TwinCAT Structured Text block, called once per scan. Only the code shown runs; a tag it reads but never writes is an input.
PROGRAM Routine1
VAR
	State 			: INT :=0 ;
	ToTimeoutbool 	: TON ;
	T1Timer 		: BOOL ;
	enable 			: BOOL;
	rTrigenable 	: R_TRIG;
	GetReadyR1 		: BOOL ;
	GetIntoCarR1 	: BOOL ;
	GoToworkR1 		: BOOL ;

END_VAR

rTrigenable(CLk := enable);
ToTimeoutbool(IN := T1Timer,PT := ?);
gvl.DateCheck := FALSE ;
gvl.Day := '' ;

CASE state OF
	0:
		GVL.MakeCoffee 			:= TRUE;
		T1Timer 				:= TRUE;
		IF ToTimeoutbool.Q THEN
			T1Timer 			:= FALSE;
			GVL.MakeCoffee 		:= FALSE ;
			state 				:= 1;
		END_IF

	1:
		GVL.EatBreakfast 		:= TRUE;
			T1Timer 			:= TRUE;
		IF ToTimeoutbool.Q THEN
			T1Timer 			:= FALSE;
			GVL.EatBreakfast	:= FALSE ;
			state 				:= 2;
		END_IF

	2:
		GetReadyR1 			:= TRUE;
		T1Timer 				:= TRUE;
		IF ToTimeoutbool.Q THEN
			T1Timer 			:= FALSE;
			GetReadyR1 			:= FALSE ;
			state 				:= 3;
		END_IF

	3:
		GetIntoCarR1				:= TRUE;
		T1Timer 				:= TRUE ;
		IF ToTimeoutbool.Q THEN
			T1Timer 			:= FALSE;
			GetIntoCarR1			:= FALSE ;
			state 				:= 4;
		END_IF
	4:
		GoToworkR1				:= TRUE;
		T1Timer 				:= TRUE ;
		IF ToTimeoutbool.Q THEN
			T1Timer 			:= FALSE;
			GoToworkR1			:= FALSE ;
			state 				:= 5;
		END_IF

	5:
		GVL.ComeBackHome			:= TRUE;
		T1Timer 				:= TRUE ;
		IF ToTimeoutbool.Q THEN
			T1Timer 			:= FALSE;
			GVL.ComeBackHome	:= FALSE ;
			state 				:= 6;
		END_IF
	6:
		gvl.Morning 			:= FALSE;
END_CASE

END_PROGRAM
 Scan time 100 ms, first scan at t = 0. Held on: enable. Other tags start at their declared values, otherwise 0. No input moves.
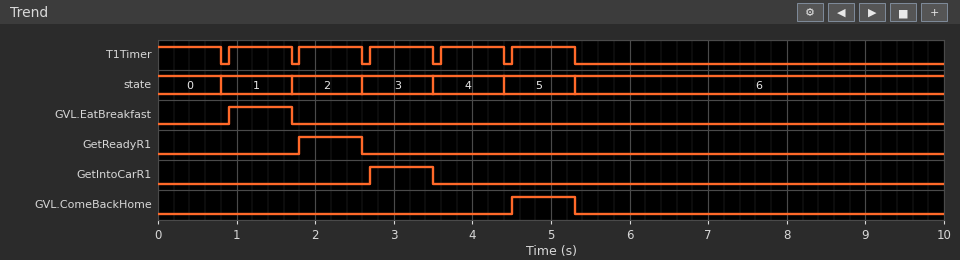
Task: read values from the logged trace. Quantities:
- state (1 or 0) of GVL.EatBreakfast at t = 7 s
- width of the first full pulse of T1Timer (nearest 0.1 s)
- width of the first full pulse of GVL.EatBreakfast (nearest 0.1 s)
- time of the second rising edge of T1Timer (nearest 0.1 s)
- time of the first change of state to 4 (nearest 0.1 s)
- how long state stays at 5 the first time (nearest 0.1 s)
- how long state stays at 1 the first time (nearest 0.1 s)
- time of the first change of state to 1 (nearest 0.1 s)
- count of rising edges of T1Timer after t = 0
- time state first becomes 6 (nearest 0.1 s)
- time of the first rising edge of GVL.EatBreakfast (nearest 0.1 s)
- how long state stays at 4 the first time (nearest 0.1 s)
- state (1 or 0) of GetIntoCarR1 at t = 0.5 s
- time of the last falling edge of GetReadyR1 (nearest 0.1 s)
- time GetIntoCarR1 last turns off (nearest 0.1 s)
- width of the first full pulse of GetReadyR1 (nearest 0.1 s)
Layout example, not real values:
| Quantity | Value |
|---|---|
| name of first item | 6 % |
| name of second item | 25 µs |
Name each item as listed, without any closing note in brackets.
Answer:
| Quantity | Value |
|---|---|
| state (1 or 0) of GVL.EatBreakfast at t = 7 s | 0 |
| width of the first full pulse of T1Timer | 0.8 s |
| width of the first full pulse of GVL.EatBreakfast | 0.8 s |
| time of the second rising edge of T1Timer | 1.8 s |
| time of the first change of state to 4 | 3.5 s |
| how long state stays at 5 the first time | 0.9 s |
| how long state stays at 1 the first time | 0.9 s |
| time of the first change of state to 1 | 0.8 s |
| count of rising edges of T1Timer after t = 0 | 5 |
| time state first becomes 6 | 5.3 s |
| time of the first rising edge of GVL.EatBreakfast | 0.9 s |
| how long state stays at 4 the first time | 0.9 s |
| state (1 or 0) of GetIntoCarR1 at t = 0.5 s | 0 |
| time of the last falling edge of GetReadyR1 | 2.6 s |
| time GetIntoCarR1 last turns off | 3.5 s |
| width of the first full pulse of GetReadyR1 | 0.8 s |
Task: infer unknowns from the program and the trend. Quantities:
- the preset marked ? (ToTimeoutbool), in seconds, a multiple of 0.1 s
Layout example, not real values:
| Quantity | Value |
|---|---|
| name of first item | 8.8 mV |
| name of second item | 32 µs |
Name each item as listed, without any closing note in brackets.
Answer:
| Quantity | Value |
|---|---|
| the preset marked ? (ToTimeoutbool), in seconds, a multiple of 0.1 s | 0.7 s |
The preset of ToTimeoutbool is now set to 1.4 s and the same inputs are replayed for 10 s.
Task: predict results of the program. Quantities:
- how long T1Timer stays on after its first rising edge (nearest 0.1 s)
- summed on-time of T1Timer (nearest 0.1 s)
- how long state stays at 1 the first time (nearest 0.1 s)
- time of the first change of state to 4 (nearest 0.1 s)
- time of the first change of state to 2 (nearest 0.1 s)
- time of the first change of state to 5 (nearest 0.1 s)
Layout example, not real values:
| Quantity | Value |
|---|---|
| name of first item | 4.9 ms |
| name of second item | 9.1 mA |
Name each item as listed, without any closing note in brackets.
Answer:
| Quantity | Value |
|---|---|
| how long T1Timer stays on after its first rising edge | 1.5 s |
| summed on-time of T1Timer | 9.0 s |
| how long state stays at 1 the first time | 1.6 s |
| time of the first change of state to 4 | 6.3 s |
| time of the first change of state to 2 | 3.1 s |
| time of the first change of state to 5 | 7.9 s |
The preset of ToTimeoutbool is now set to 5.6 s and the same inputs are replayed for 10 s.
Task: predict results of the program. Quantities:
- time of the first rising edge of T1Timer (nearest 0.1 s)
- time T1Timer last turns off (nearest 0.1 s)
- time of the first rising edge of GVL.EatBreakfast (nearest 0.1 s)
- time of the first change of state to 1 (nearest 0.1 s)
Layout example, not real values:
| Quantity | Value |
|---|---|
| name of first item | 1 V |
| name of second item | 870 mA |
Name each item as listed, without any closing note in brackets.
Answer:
| Quantity | Value |
|---|---|
| time of the first rising edge of T1Timer | 5.8 s |
| time T1Timer last turns off | 5.7 s |
| time of the first rising edge of GVL.EatBreakfast | 5.8 s |
| time of the first change of state to 1 | 5.7 s |
